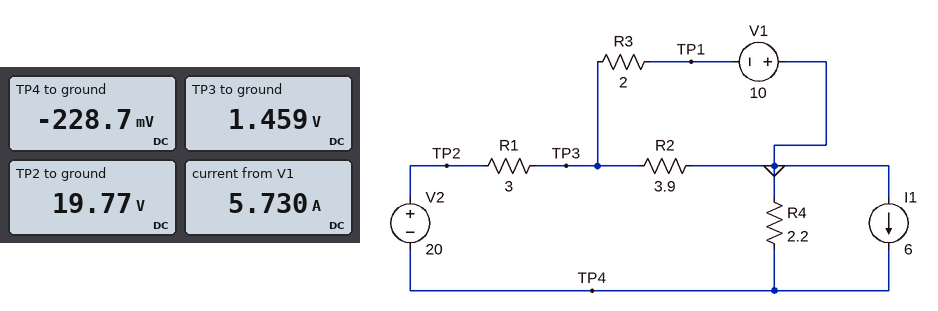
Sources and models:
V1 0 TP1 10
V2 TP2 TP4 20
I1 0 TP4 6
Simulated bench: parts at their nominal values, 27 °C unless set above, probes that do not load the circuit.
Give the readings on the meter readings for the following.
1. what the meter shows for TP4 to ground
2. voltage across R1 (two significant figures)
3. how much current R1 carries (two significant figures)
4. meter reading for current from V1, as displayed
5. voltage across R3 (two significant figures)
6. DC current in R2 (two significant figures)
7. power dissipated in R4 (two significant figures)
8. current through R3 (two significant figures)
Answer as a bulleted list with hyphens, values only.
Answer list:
- -228.7 mV
- 18 V
- 6.1 A
- 5.730 A
- 11 V
- 370 mA
- 24 mW
- 5.7 A
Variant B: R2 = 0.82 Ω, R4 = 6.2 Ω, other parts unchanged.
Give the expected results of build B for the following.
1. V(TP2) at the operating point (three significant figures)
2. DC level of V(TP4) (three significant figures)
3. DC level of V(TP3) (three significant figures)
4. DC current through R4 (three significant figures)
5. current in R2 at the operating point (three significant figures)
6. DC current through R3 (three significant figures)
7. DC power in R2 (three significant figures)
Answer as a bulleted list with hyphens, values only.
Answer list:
- 19.1 V
- -899 mV
- 666 mV
- 145 mA
- 812 mA
- 5.33 A
- 541 mW
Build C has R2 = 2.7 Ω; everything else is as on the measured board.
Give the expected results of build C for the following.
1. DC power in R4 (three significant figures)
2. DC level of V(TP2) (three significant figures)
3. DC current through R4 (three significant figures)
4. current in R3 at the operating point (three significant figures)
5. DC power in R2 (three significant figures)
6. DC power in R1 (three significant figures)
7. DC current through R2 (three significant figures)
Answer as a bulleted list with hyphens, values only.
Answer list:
- 39.5 mW
- 19.7 V
- 134 mA
- 5.65 A
- 629 mW
- 113 W
- 483 mA
